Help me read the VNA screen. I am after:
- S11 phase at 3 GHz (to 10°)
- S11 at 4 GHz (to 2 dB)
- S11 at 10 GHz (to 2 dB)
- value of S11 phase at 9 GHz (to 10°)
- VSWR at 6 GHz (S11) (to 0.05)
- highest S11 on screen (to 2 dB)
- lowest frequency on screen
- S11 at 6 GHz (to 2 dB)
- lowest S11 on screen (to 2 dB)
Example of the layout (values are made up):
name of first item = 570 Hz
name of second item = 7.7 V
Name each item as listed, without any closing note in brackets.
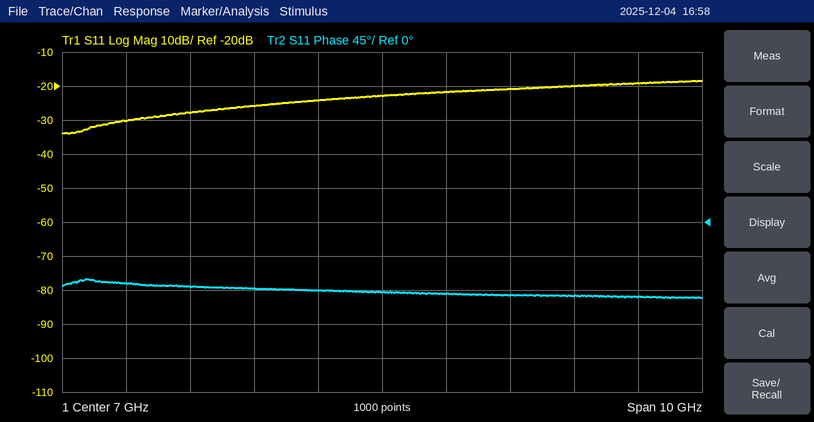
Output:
S11 phase at 3 GHz = -80°
S11 at 4 GHz = -28 dB
S11 at 10 GHz = -20 dB
value of S11 phase at 9 GHz = -100°
VSWR at 6 GHz (S11) = 1.15
highest S11 on screen = -18 dB
lowest frequency on screen = 2 GHz
S11 at 6 GHz = -24 dB
lowest S11 on screen = -34 dB
